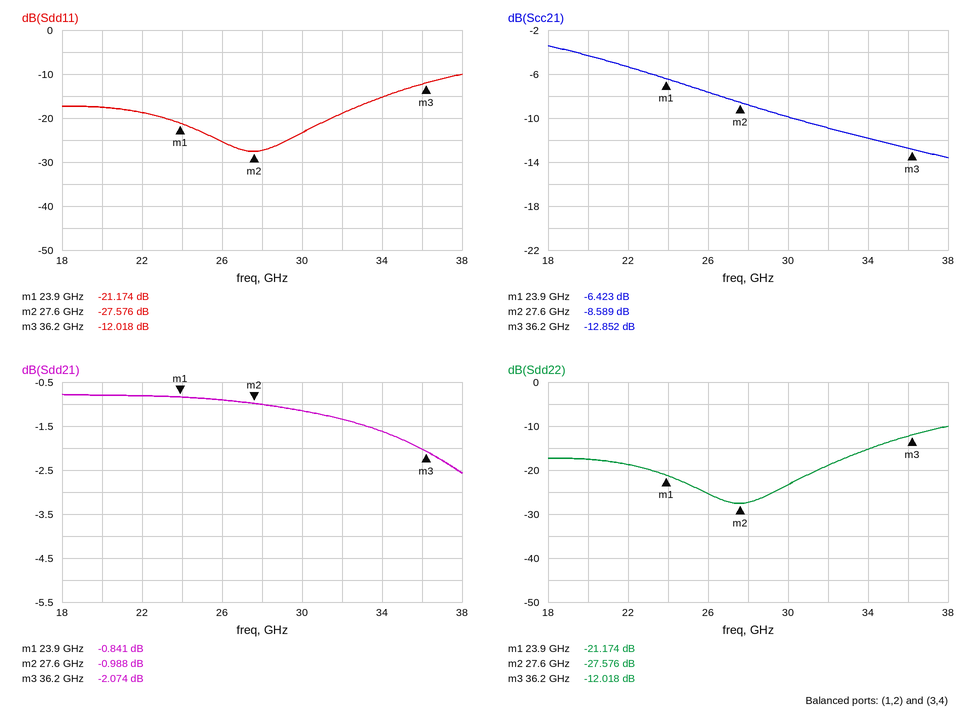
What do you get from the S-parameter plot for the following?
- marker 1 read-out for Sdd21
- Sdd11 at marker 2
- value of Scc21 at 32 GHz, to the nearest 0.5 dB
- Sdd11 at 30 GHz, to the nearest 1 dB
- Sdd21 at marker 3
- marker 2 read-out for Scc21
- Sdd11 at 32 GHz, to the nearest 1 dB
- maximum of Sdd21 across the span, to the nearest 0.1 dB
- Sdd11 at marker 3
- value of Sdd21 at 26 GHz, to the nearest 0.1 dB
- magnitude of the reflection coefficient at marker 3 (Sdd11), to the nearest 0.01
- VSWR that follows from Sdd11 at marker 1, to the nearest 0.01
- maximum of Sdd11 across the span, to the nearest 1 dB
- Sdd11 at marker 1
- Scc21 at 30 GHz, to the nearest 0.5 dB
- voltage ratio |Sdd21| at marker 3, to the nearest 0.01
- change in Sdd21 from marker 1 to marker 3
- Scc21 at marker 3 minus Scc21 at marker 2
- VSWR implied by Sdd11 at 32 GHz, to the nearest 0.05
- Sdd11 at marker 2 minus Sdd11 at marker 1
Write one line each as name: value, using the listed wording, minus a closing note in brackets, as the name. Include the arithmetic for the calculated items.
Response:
marker 1 read-out for Sdd21: -0.841 dB
Sdd11 at marker 2: -27.576 dB
value of Scc21 at 32 GHz, to the nearest 0.5 dB: -11.0 dB
Sdd11 at 30 GHz, to the nearest 1 dB: -23 dB
Sdd21 at marker 3: -2.074 dB
marker 2 read-out for Scc21: -8.589 dB
Sdd11 at 32 GHz, to the nearest 1 dB: -19 dB
maximum of Sdd21 across the span, to the nearest 0.1 dB: -0.8 dB
Sdd11 at marker 3: -12.018 dB
value of Sdd21 at 26 GHz, to the nearest 0.1 dB: -0.9 dB
magnitude of the reflection coefficient at marker 3 (Sdd11), to the nearest 0.01: 10^(-12.018/20) ≈ 0.25
VSWR that follows from Sdd11 at marker 1, to the nearest 0.01: (1 + 0.0874)/(1 − 0.0874) ≈ 1.19
maximum of Sdd11 across the span, to the nearest 1 dB: -10 dB
Sdd11 at marker 1: -21.174 dB
Scc21 at 30 GHz, to the nearest 0.5 dB: -10.0 dB
voltage ratio |Sdd21| at marker 3, to the nearest 0.01: 10^(-2.074/20) ≈ 0.79
change in Sdd21 from marker 1 to marker 3: -2.074 − (-0.841) = -1.233 dB
Scc21 at marker 3 minus Scc21 at marker 2: -12.852 − (-8.589) = -4.263 dB
VSWR implied by Sdd11 at 32 GHz, to the nearest 0.05: |Γ| = 10^(-19/20) = 0.1122; VSWR = (1 + 0.1122)/(1 − 0.1122) ≈ 1.25
Sdd11 at marker 2 minus Sdd11 at marker 1: -27.576 − (-21.174) = -6.402 dB
